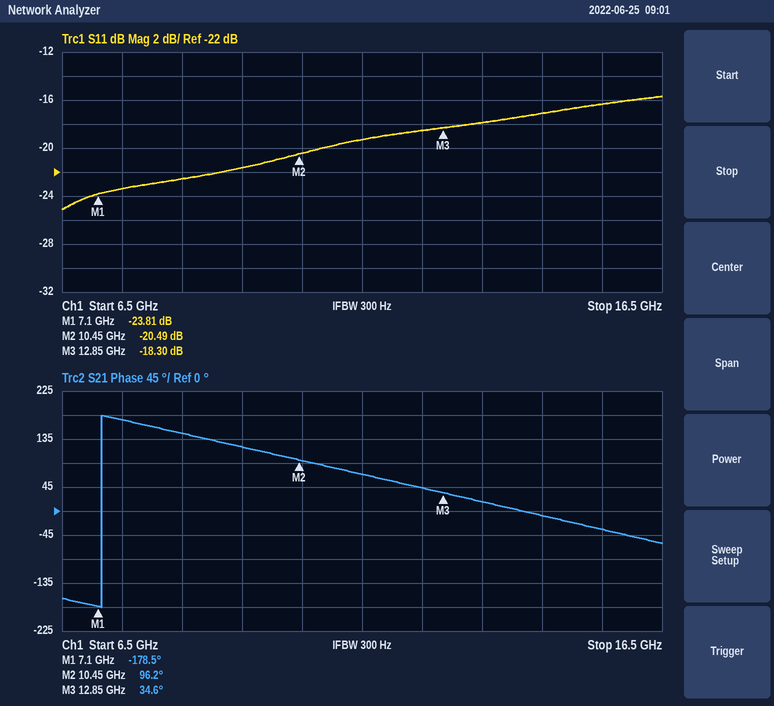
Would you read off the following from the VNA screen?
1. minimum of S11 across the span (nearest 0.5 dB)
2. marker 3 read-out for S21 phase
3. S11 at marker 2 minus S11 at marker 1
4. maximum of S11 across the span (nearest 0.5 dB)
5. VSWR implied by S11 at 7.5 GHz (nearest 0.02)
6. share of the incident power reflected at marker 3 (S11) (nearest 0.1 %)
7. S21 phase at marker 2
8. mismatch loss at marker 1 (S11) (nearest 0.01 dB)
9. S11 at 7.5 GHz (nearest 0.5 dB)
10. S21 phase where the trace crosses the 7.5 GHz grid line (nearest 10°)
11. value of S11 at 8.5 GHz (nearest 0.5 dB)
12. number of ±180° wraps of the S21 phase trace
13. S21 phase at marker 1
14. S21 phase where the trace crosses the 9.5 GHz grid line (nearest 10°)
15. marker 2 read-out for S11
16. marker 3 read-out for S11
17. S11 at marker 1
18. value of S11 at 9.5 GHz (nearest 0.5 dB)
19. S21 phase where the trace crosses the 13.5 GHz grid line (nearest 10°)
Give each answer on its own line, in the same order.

-25.0 dB
34.6°
3.32 dB
-15.5 dB
1.14
1.5 %
96.2°
0.02 dB
-23.5 dB
170°
-22.5 dB
1
-178.5°
120°
-20.49 dB
-18.30 dB
-23.81 dB
-21.5 dB
20°
